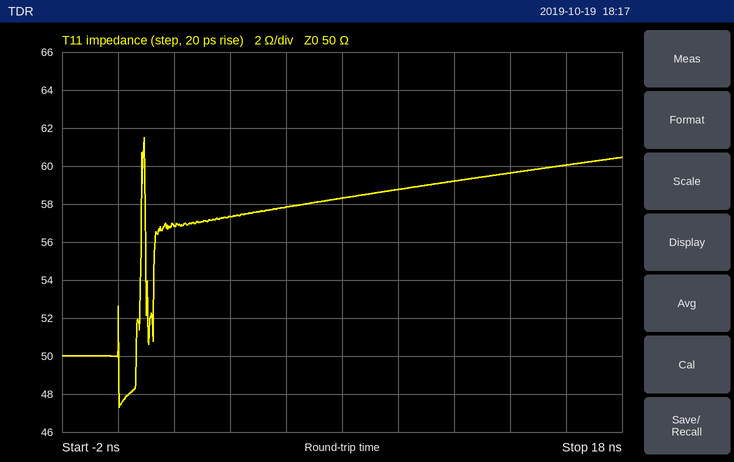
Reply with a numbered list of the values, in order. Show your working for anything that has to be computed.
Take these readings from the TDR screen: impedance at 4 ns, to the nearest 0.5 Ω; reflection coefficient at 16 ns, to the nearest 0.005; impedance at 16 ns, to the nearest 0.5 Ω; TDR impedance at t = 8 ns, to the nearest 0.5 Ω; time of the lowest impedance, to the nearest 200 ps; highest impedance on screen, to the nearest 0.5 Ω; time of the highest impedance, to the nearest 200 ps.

1. 57.5 Ω
2. (60 − 50)/(60 + 50) ≈ +0.0909, so +0.090 to the nearest 0.005
3. 60.0 Ω
4. 58.5 Ω
5. 0.0 ns
6. 61.5 Ω
7. 1.0 ns
